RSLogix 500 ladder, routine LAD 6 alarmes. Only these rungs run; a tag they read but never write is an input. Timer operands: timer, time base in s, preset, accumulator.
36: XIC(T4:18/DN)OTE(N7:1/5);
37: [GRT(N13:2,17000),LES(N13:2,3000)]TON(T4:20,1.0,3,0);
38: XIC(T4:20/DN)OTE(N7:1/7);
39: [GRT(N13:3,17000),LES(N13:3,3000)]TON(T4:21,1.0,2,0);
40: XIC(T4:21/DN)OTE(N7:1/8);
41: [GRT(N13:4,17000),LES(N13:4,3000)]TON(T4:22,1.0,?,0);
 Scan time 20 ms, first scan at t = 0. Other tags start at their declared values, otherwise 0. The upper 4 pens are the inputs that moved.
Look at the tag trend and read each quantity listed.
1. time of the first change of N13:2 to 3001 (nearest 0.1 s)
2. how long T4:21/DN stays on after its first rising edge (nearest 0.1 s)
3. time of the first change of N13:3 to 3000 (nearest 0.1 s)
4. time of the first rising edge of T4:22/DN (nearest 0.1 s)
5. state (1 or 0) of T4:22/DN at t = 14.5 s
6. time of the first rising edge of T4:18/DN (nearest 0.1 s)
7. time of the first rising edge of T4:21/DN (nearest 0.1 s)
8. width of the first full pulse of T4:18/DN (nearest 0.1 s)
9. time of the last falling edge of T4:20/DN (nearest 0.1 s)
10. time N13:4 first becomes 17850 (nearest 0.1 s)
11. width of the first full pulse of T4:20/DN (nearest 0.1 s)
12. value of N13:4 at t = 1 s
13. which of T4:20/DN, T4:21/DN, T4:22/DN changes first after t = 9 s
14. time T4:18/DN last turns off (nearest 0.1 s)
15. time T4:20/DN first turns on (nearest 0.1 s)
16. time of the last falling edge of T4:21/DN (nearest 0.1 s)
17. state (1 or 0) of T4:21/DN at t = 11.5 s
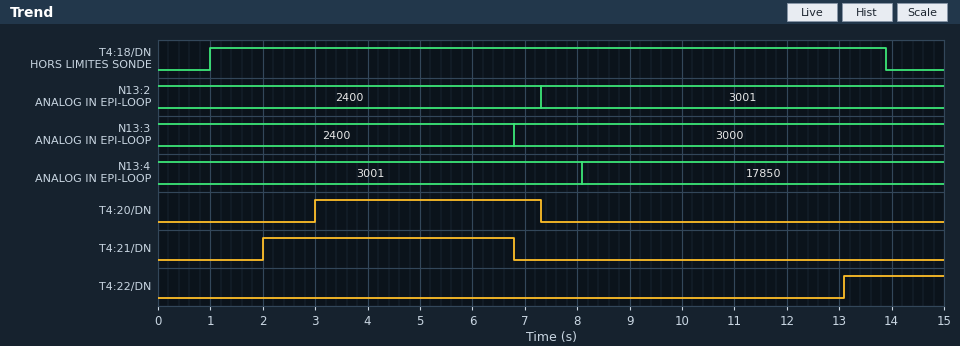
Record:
7.3 s
4.8 s
6.8 s
13.1 s
1
1.0 s
2.0 s
12.9 s
7.3 s
8.1 s
4.3 s
3001
T4:22/DN
13.9 s
3.0 s
6.8 s
0
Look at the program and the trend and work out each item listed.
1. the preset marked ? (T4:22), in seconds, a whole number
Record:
5 s
